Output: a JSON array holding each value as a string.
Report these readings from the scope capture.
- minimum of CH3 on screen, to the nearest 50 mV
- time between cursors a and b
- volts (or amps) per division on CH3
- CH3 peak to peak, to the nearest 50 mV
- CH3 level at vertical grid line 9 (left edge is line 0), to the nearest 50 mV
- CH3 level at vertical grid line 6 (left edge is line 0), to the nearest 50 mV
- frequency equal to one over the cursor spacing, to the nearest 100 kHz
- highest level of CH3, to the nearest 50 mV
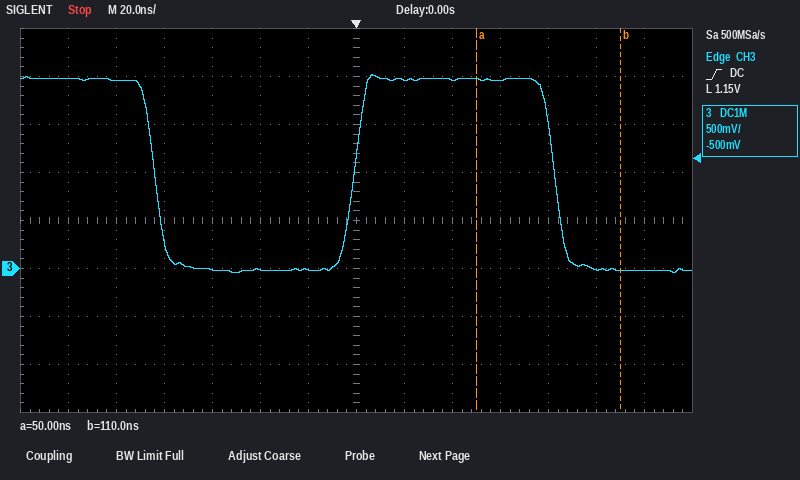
["-50 mV", "60 ns", "500 mV", "2.05 V", "1.95 V", "0 mV", "16.7 MHz", "2.00 V"]
